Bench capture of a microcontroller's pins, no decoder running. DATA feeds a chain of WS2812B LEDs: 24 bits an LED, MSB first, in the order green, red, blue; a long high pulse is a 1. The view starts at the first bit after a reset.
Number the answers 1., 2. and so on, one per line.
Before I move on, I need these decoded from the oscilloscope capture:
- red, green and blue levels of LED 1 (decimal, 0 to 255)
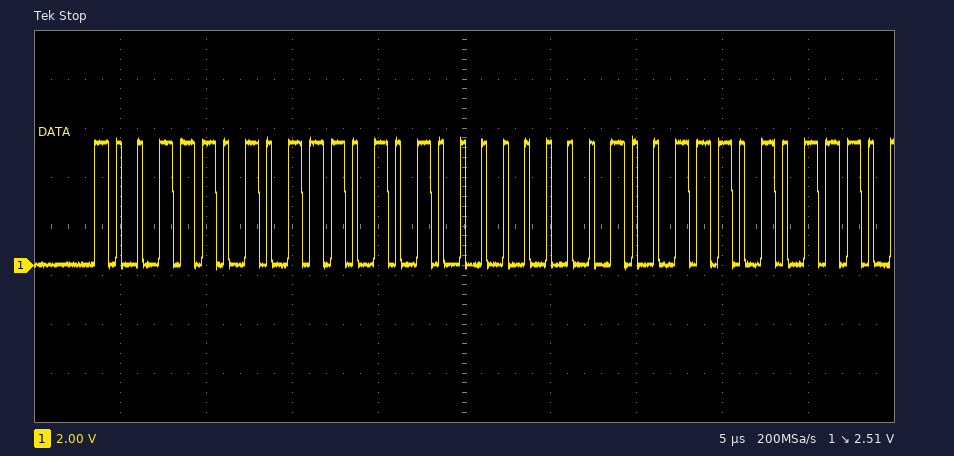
1. 117, 157, 0
